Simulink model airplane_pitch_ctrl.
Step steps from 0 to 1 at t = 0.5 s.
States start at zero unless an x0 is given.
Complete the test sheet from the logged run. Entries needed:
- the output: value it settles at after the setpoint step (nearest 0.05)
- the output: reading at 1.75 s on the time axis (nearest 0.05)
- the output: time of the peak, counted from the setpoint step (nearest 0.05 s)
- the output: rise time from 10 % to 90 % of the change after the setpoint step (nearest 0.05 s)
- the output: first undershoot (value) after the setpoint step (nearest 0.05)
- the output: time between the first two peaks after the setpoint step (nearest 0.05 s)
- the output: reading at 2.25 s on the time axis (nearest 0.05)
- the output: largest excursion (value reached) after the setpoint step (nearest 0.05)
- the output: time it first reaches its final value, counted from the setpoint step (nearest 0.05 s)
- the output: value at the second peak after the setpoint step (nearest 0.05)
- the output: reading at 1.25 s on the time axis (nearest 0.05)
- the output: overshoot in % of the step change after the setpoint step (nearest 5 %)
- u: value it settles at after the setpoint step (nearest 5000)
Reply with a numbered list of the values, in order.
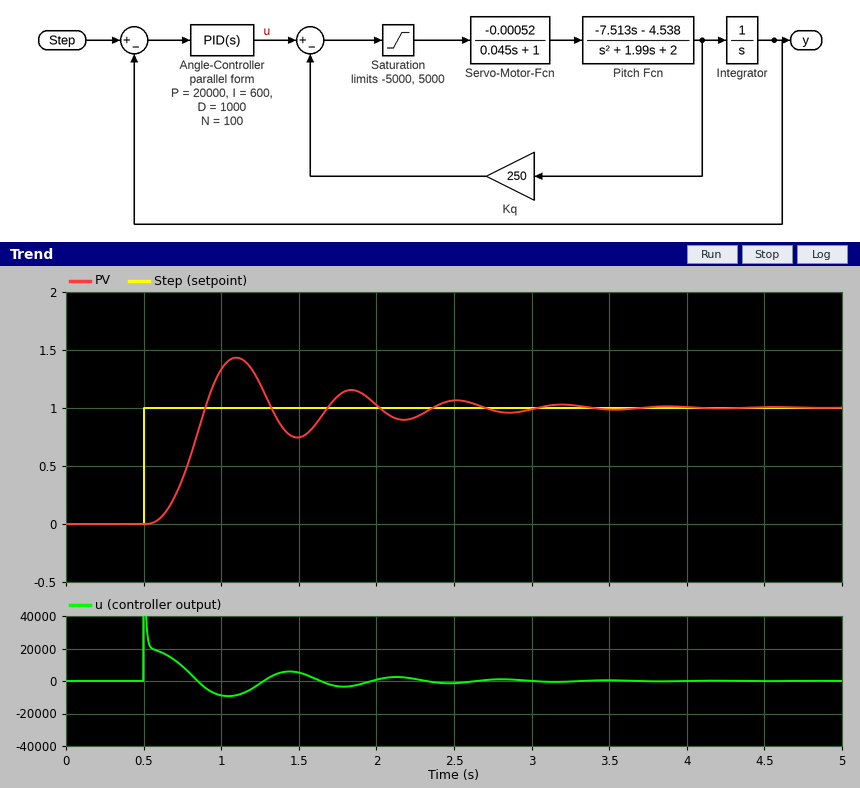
1. 1.00
2. 1.10
3. 0.60 s
4. 0.25 s
5. 0.75
6. 0.75 s
7. 0.90
8. 1.45
9. 0.40 s
10. 1.15
11. 1.20
12. 45 %
13. 0
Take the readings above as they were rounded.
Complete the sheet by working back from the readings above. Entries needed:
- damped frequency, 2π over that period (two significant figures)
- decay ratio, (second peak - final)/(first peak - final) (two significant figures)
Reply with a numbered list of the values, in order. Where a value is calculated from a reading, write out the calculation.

1. 2π / 0.75 = 8.4 rad/s
2. (1.15 - 1) / (1.45 - 1) = 0.33
